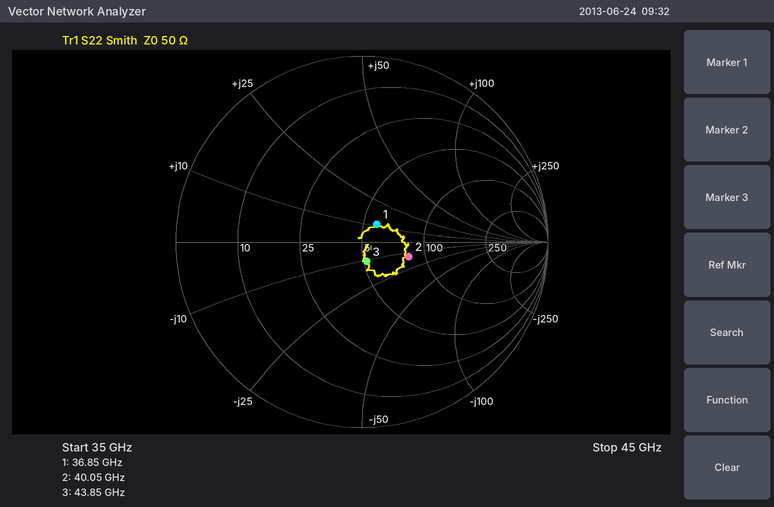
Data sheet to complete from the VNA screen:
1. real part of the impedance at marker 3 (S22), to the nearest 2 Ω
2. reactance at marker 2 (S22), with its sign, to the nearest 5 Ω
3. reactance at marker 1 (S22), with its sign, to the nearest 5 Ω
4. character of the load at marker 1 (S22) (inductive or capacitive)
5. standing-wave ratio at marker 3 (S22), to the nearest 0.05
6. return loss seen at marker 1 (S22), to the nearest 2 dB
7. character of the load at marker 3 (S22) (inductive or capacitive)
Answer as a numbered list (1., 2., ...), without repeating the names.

1. 52 Ω
2. -15 Ω
3. +10 Ω
4. inductive
5. 1.25
6. 18 dB
7. capacitive
